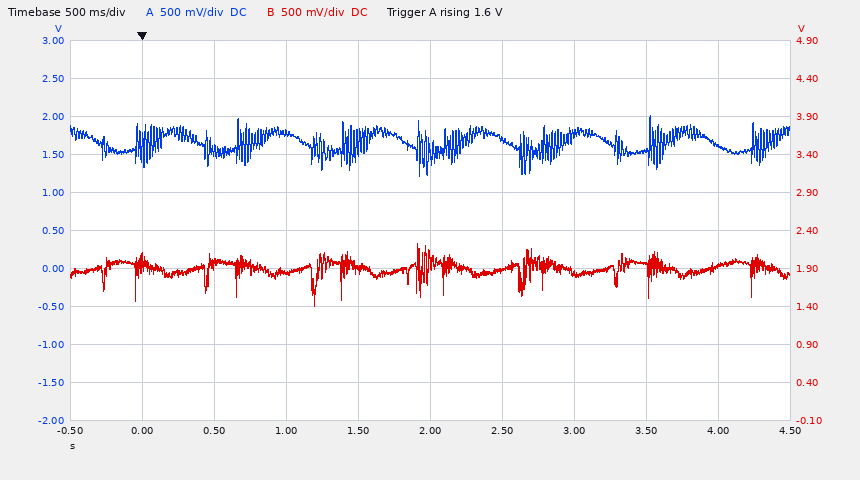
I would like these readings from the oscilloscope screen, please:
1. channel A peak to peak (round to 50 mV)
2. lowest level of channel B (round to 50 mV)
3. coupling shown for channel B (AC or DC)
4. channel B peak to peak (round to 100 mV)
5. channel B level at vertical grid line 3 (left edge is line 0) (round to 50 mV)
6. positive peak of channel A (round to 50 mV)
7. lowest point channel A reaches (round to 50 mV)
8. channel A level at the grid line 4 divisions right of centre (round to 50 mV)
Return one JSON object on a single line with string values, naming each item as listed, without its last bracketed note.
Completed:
{"channel A peak to peak": "800 mV", "lowest level of channel B": "1.40 V", "coupling shown for channel B": "DC", "channel B peak to peak": "800 mV", "channel B level at vertical grid line 3 (left edge is line 0)": "1.85 V", "positive peak of channel A": "2.00 V", "lowest point channel A reaches": "1.20 V", "channel A level at the grid line 4 divisions right of centre": "1.60 V"}
